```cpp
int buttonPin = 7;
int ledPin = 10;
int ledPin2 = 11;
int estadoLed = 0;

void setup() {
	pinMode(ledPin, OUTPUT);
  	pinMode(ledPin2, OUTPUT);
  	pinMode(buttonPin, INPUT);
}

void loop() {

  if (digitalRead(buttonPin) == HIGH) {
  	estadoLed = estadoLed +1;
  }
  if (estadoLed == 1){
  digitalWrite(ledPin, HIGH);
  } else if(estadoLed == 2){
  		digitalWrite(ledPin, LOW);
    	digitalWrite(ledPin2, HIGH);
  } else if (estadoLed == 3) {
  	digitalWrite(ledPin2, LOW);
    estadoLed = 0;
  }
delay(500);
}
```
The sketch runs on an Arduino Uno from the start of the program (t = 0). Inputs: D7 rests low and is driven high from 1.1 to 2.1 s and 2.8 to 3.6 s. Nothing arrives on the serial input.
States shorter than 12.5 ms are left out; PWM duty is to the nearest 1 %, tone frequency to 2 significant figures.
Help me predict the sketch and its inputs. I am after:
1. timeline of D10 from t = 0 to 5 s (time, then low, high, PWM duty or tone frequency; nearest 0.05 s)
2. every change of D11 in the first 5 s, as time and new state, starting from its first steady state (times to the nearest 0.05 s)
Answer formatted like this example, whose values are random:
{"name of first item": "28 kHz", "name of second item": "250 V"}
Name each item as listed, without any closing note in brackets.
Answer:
{"timeline of D10 from t = 0 to 5 s": "0 s low; 1.5 s high; 2 s low; 3.5 s high", "every change of D11 in the first 5 s, as time and new state, starting from its first steady state": "0 s low; 2 s high; 3 s low"}
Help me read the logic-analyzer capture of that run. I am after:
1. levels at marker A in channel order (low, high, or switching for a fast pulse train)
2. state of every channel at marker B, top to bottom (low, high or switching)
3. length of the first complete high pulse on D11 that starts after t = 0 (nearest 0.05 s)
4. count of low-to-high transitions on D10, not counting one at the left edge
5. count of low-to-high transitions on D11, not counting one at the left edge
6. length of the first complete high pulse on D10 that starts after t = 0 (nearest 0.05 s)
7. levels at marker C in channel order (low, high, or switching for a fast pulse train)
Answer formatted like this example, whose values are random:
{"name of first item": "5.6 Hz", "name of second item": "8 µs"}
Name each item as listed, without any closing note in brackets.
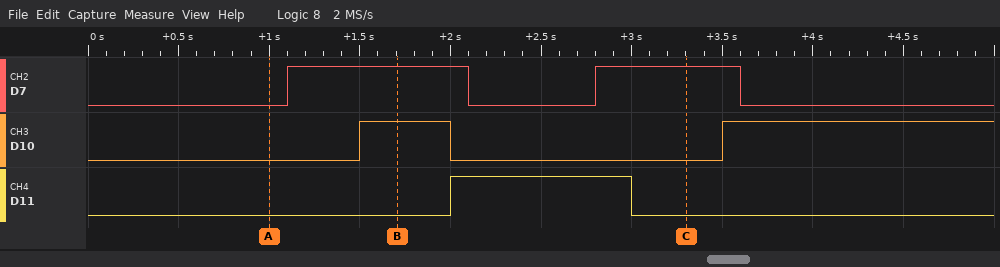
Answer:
{"levels at marker A in channel order": "D7 low, D10 low, D11 low", "state of every channel at marker B, top to bottom": "D7 high, D10 high, D11 low", "length of the first complete high pulse on D11 that starts after t = 0": "1.00 s", "count of low-to-high transitions on D10, not counting one at the left edge": "2", "count of low-to-high transitions on D11, not counting one at the left edge": "1", "length of the first complete high pulse on D10 that starts after t = 0": "0.50 s", "levels at marker C in channel order": "D7 high, D10 low, D11 low"}
